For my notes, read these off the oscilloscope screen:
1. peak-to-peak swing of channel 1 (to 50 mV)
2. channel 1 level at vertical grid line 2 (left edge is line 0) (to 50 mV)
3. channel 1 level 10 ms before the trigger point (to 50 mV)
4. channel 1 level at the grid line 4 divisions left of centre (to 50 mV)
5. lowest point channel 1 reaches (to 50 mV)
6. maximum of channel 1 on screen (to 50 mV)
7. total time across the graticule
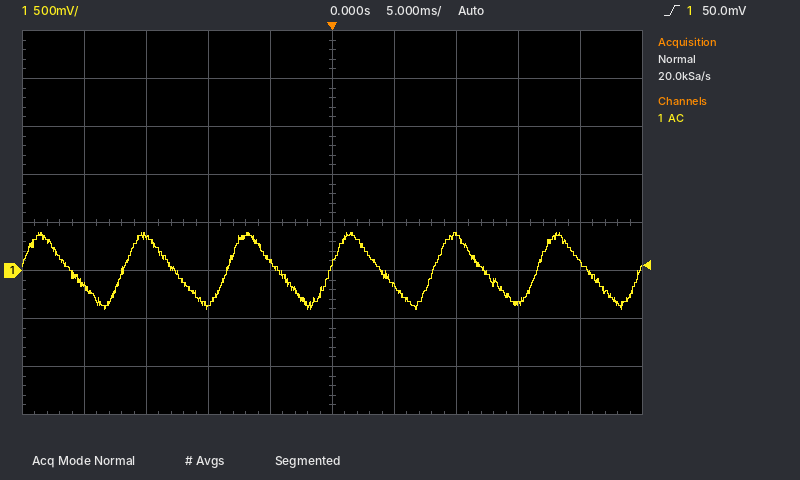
800 mV
350 mV
-350 mV
-150 mV
-400 mV
400 mV
50 ms
